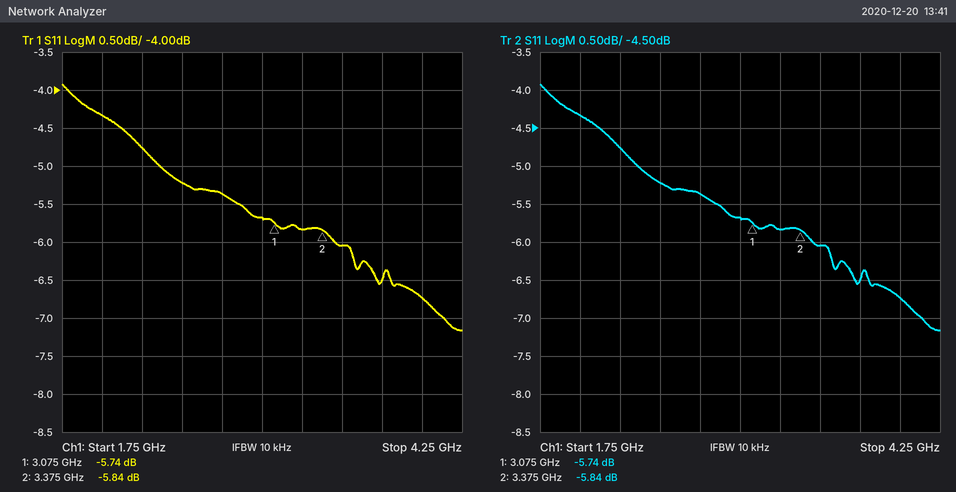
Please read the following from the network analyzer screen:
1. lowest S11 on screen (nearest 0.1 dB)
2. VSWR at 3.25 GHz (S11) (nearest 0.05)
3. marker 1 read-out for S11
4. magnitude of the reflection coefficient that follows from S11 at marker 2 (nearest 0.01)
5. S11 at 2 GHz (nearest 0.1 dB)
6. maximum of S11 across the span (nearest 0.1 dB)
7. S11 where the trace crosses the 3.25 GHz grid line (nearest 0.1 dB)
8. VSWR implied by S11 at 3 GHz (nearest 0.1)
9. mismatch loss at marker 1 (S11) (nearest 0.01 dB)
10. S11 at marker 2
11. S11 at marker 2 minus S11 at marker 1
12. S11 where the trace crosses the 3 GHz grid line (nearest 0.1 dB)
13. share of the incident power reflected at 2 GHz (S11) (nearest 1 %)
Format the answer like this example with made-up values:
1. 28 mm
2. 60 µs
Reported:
1. -7.2 dB
2. 3.10
3. -5.74 dB
4. 0.51
5. -4.3 dB
6. -3.9 dB
7. -5.8 dB
8. 3.2
9. 1.35 dB
10. -5.84 dB
11. -0.10 dB
12. -5.7 dB
13. 37 %
